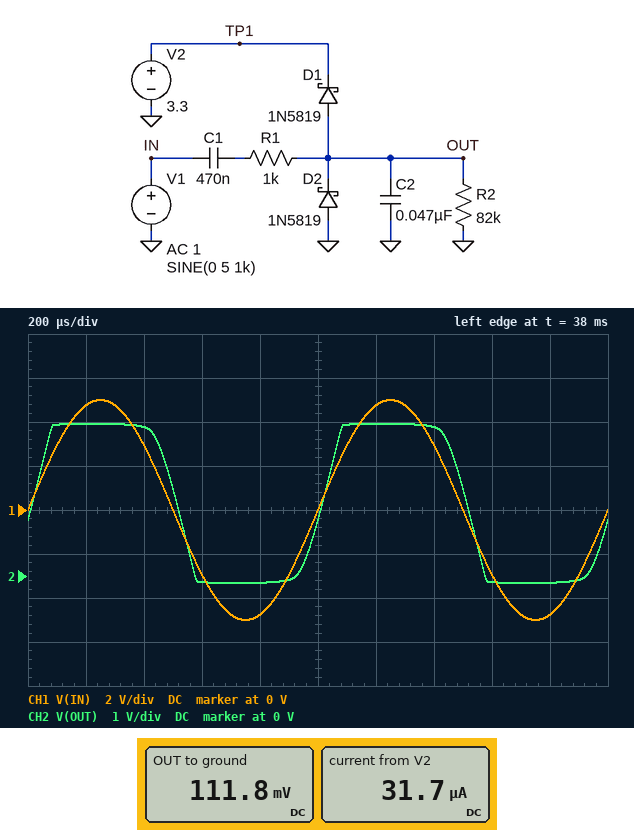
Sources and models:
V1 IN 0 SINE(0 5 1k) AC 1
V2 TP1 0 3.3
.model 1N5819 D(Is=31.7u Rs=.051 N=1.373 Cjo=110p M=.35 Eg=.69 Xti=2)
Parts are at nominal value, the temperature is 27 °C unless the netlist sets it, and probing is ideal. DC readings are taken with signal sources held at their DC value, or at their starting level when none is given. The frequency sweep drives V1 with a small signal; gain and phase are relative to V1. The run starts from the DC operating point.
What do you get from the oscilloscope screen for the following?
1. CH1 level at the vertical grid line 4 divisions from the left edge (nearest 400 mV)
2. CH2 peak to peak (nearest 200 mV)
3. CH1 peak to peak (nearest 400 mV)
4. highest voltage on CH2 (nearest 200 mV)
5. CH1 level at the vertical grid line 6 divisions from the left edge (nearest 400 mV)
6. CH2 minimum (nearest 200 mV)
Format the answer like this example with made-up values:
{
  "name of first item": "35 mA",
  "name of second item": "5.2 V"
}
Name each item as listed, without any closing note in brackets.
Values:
{
  "CH1 level at the vertical grid line 4 divisions from the left edge": "-4.8 V",
  "CH2 peak to peak": "3.6 V",
  "CH1 peak to peak": "10.0 V",
  "highest voltage on CH2": "3.4 V",
  "CH1 level at the vertical grid line 6 divisions from the left edge": "4.8 V",
  "CH2 minimum": "-200 mV"
}
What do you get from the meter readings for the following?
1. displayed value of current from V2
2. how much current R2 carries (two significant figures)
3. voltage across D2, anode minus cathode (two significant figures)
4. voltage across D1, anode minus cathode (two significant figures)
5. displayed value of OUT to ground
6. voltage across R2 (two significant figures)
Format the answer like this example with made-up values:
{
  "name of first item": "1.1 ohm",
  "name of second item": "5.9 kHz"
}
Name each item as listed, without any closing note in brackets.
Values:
{
  "displayed value of current from V2": "31.7 µA",
  "how much current R2 carries": "1.4 µA",
  "voltage across D2, anode minus cathode": "-110 mV",
  "voltage across D1, anode minus cathode": "-3.2 V",
  "displayed value of OUT to ground": "111.8 mV",
  "voltage across R2": "110 mV"
}
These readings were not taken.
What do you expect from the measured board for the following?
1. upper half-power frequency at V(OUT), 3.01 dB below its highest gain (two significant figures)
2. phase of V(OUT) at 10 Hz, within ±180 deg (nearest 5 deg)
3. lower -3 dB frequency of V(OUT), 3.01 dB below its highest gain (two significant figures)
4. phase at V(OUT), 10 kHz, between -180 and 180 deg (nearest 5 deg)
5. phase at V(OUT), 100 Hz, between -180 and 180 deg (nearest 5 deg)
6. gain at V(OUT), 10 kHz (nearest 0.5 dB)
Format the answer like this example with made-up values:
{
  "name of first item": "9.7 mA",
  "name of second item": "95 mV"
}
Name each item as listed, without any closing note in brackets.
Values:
{
  "upper half-power frequency at V(OUT), 3.01 dB below its highest gain": "3.9 kHz",
  "phase of V(OUT) at 10 Hz, within ±180 deg": "55 deg",
  "lower -3 dB frequency of V(OUT), 3.01 dB below its highest gain": "14 Hz",
  "phase at V(OUT), 10 kHz, between -180 and 180 deg": "-70 deg",
  "phase at V(OUT), 100 Hz, between -180 and 180 deg": "5 deg",
  "gain at V(OUT), 10 kHz": "-10.0 dB"
}
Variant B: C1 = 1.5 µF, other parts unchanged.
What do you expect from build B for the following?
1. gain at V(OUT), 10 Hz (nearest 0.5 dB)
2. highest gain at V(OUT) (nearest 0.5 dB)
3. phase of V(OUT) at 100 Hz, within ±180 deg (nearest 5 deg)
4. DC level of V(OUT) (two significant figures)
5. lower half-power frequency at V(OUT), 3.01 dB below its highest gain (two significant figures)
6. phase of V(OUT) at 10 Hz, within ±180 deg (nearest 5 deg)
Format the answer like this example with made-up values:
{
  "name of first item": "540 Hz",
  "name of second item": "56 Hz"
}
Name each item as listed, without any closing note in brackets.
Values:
{
  "gain at V(OUT), 10 Hz": "-1.5 dB",
  "highest gain at V(OUT)": "-0.5 dB",
  "phase of V(OUT) at 100 Hz, within ±180 deg": "0 deg",
  "DC level of V(OUT)": "110 mV",
  "lower half-power frequency at V(OUT), 3.01 dB below its highest gain": "4.8 Hz",
  "phase of V(OUT) at 10 Hz, within ±180 deg": "25 deg"
}
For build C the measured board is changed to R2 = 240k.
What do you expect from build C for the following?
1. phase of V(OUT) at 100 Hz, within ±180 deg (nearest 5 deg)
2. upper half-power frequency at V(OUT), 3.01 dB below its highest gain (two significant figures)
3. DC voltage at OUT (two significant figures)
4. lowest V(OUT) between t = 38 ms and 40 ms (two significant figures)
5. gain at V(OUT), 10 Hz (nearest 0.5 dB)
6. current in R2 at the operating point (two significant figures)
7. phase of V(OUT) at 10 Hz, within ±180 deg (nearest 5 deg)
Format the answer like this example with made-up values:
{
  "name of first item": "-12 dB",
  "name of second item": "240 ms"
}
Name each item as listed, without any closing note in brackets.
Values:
{
  "phase of V(OUT) at 100 Hz, within ±180 deg": "0 deg",
  "upper half-power frequency at V(OUT), 3.01 dB below its highest gain": "3.8 kHz",
  "DC voltage at OUT": "150 mV",
  "lowest V(OUT) between t = 38 ms and 40 ms": "-160 mV",
  "gain at V(OUT), 10 Hz": "-2.0 dB",
  "current in R2 at the operating point": "610 nA",
  "phase of V(OUT) at 10 Hz, within ±180 deg": "25 deg"
}
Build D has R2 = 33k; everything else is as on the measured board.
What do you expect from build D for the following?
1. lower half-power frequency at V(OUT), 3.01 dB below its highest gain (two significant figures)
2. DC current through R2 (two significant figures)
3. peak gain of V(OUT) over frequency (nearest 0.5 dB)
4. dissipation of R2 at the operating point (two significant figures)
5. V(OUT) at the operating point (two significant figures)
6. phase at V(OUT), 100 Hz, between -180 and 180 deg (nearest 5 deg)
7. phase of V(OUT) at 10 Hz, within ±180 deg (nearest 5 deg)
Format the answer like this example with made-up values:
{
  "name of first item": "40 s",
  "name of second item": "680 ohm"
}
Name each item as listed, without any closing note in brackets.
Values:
{
  "lower half-power frequency at V(OUT), 3.01 dB below its highest gain": "29 Hz",
  "DC current through R2": "2.7 µA",
  "peak gain of V(OUT) over frequency": "-1.5 dB",
  "dissipation of R2 at the operating point": "230 nW",
  "V(OUT) at the operating point": "88 mV",
  "phase at V(OUT), 100 Hz, between -180 and 180 deg": "15 deg",
  "phase of V(OUT) at 10 Hz, within ±180 deg": "70 deg"
}
